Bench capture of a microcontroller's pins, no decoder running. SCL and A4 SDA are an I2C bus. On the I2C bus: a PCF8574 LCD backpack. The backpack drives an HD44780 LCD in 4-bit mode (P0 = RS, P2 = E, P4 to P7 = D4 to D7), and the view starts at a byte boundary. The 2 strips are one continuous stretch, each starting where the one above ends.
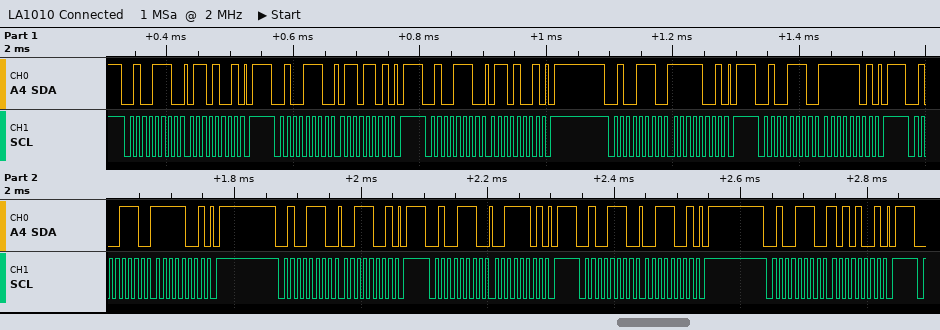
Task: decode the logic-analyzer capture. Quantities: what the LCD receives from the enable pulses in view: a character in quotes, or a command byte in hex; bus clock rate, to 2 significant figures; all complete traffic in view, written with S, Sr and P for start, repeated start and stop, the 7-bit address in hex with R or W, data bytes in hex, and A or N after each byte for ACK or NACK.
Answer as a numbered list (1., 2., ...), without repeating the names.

1. 'o'
2. 100 kHz
3. S 27W A 69 A P S 27W A 6D A P S 27W A 69 A P S 27W A F9 A P S 27W A FD A P S 27W A F9 A P S 27W A 39 A P S 27W A 3D A P S 27W A 39 A P S 27W A A9 A P
